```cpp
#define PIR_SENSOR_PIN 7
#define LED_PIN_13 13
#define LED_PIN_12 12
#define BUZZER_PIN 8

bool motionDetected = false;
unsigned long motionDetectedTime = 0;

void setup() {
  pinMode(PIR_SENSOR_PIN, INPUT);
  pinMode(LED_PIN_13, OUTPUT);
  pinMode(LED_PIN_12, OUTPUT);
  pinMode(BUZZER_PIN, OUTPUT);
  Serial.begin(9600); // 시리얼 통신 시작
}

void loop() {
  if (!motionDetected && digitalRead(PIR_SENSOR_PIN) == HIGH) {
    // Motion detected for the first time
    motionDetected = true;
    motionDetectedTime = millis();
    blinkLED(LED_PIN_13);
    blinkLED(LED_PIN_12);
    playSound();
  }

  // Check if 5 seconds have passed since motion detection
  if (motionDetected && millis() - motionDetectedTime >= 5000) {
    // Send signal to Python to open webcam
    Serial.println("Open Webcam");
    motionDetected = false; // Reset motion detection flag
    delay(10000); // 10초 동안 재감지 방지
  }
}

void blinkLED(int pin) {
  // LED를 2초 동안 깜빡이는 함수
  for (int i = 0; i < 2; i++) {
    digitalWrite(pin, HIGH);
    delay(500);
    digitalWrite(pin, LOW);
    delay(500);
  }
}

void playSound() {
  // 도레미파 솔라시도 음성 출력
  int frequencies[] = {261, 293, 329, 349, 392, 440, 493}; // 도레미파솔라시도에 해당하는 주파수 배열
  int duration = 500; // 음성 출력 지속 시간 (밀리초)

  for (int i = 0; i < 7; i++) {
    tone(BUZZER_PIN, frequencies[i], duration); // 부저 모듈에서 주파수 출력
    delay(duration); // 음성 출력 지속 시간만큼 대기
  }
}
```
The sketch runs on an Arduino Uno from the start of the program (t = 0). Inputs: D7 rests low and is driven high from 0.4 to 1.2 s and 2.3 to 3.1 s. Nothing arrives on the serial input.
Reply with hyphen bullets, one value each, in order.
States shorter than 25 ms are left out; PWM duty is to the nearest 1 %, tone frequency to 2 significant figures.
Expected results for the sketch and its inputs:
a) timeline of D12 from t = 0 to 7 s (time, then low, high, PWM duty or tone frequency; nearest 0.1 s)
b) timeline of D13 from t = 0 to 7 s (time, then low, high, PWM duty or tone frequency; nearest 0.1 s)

- 0 s low; 2.4 s high; 2.9 s low; 3.4 s high; 3.9 s low
- 0 s low; 0.4 s high; 0.9 s low; 1.4 s high; 1.9 s low
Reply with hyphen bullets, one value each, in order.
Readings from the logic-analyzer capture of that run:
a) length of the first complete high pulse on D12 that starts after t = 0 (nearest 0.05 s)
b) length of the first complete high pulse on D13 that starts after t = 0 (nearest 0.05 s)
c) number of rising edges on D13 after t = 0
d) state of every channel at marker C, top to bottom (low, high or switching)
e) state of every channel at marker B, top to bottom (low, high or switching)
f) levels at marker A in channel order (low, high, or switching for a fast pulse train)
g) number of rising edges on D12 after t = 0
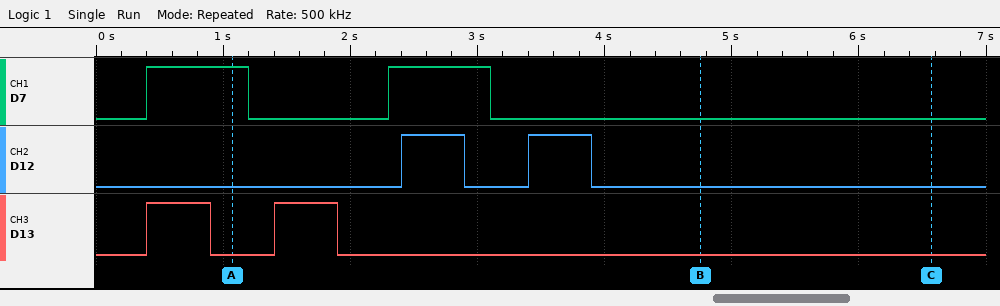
- 0.50 s
- 0.50 s
- 2
- D7 low, D12 low, D13 low
- D7 low, D12 low, D13 low
- D7 high, D12 low, D13 low
- 2
